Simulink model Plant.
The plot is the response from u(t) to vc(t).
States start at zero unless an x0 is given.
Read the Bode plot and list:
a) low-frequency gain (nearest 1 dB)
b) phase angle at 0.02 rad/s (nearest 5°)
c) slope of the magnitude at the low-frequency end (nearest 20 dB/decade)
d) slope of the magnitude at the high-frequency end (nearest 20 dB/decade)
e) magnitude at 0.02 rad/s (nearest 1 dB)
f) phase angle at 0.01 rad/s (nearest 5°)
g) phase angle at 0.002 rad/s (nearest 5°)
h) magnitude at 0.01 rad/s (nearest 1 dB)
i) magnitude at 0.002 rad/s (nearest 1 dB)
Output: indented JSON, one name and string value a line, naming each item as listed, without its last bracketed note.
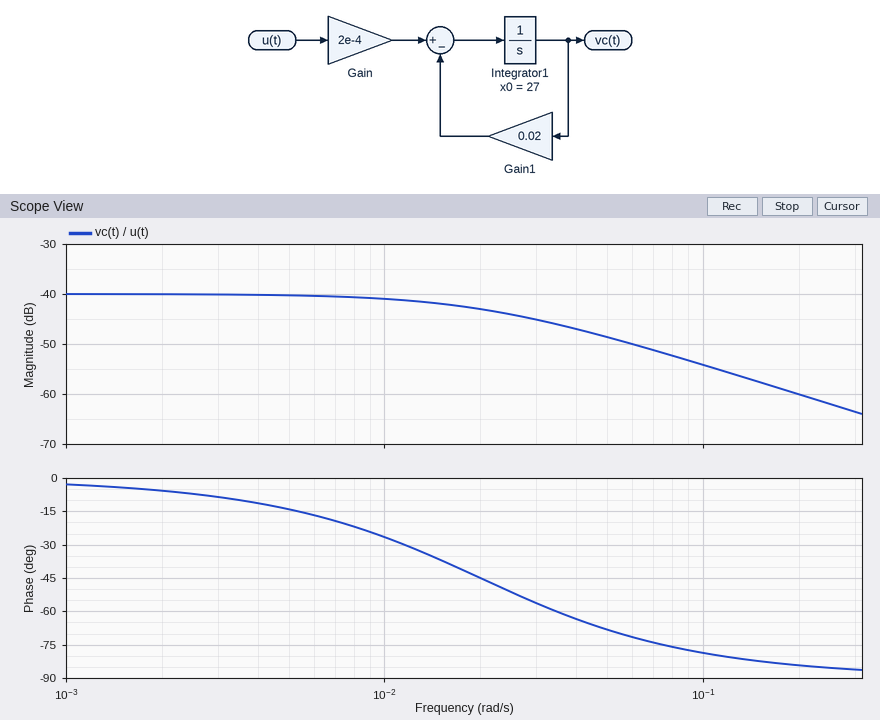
{
  "low-frequency gain": "-40 dB",
  "phase angle at 0.02 rad/s": "-45°",
  "slope of the magnitude at the low-frequency end": "0 dB/decade",
  "slope of the magnitude at the high-frequency end": "-20 dB/decade",
  "magnitude at 0.02 rad/s": "-43 dB",
  "phase angle at 0.01 rad/s": "-25°",
  "phase angle at 0.002 rad/s": "-5°",
  "magnitude at 0.01 rad/s": "-41 dB",
  "magnitude at 0.002 rad/s": "-40 dB"
}
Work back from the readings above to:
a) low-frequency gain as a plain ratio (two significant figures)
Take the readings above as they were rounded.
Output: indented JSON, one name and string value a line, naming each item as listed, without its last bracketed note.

{
  "low-frequency gain as a plain ratio": "0.010"
}
